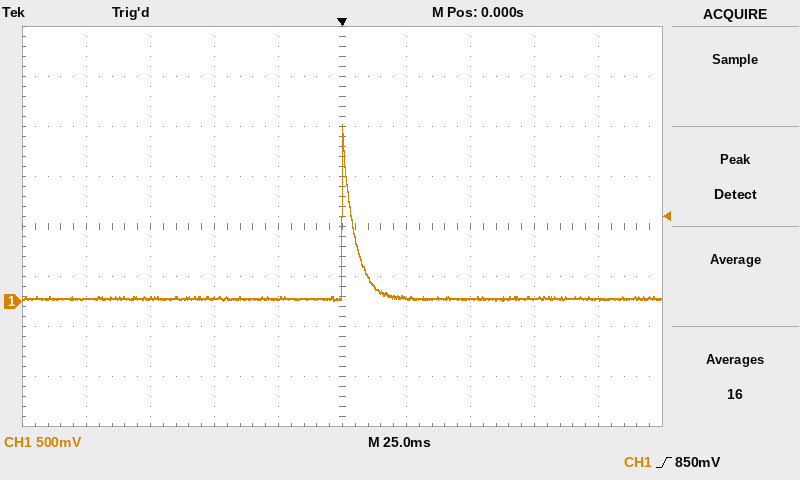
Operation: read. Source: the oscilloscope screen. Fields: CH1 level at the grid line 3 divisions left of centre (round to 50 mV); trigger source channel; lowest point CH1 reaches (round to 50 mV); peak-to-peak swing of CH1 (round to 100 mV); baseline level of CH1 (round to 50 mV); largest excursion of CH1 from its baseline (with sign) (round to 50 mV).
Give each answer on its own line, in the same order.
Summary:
50 mV
CH1
0 mV
1.80 V
50 mV
+1.75 V
